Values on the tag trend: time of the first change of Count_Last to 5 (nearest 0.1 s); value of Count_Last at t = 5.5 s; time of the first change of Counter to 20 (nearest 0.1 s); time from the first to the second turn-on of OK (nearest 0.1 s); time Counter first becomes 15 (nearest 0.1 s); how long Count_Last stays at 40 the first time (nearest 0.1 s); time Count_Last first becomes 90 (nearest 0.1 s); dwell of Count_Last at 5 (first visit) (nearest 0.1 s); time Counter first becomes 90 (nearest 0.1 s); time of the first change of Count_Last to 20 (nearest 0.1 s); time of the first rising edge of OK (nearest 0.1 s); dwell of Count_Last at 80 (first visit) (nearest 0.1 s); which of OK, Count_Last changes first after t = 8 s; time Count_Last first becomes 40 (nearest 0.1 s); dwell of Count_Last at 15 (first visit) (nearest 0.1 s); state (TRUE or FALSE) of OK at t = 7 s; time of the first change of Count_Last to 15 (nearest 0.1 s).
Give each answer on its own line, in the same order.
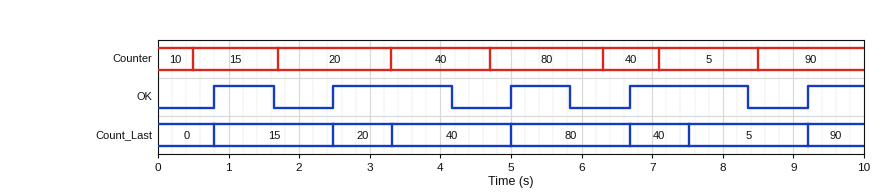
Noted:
7.5 s
80
1.7 s
1.7 s
0.5 s
1.7 s
9.2 s
1.7 s
8.5 s
2.5 s
0.8 s
1.7 s
OK
3.3 s
1.7 s
TRUE
0.8 s
